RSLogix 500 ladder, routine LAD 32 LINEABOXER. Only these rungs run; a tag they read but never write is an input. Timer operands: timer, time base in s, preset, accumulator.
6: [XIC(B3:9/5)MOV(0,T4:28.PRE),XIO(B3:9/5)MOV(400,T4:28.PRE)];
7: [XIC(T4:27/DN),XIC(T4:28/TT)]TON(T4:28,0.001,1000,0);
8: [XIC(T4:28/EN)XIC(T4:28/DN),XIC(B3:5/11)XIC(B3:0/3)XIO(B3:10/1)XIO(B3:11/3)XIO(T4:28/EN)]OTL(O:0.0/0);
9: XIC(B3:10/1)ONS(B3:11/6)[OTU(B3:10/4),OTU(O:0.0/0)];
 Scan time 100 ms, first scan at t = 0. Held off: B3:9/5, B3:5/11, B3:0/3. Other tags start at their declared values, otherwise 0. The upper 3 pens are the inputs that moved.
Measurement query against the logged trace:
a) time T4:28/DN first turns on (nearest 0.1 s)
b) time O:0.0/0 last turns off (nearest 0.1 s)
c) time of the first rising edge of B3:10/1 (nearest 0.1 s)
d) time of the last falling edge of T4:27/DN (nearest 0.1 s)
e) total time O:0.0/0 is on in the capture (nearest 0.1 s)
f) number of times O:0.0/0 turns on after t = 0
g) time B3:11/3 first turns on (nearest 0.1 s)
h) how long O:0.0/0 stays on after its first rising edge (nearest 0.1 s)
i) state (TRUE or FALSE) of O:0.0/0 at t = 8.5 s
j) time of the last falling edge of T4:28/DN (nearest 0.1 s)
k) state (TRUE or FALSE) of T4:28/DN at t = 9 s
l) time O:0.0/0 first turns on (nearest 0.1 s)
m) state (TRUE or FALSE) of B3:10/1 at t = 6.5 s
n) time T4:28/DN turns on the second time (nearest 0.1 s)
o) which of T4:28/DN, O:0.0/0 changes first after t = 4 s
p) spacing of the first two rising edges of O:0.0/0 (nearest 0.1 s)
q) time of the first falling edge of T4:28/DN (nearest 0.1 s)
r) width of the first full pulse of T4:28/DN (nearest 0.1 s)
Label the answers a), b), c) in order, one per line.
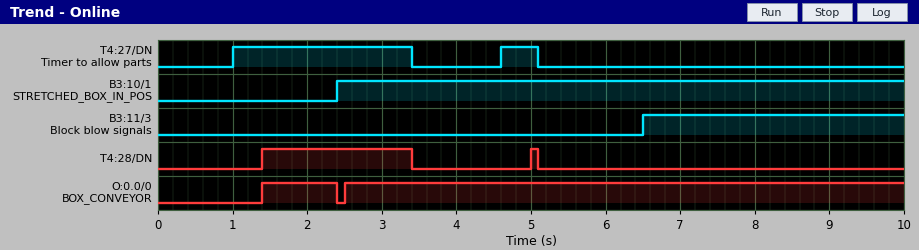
a) 1.4 s
b) 2.4 s
c) 2.4 s
d) 5.1 s
e) 8.5 s
f) 2
g) 6.5 s
h) 1.0 s
i) TRUE
j) 5.1 s
k) FALSE
l) 1.4 s
m) TRUE
n) 5.0 s
o) T4:28/DN
p) 1.1 s
q) 3.4 s
r) 2.0 s
